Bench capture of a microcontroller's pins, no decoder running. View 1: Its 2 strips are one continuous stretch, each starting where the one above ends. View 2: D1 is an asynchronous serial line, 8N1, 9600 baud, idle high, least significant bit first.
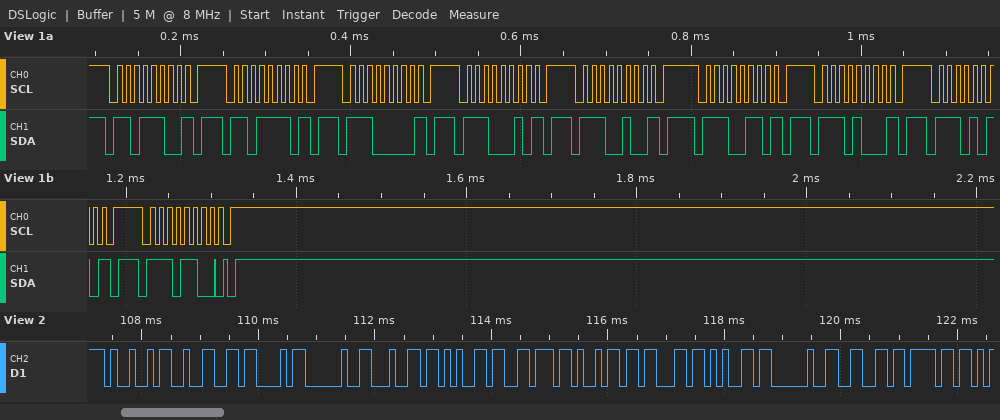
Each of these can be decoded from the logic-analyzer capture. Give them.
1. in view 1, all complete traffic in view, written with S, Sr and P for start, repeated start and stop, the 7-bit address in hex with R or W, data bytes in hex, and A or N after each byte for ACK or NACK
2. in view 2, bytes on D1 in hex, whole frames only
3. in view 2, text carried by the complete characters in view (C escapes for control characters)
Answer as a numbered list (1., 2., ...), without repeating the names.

1. S 6EW N P S 6FW N P S 70W N P S 71W N P S 72W N P S 73W N P S 74W N P S 75W N P S 76W A P
2. 0x49 0x32 0x43 0x20 0x64 0x65 0x76 0x69 0x63 0x65 0x20 0x66 0x6F
3. "I2C device fo"
